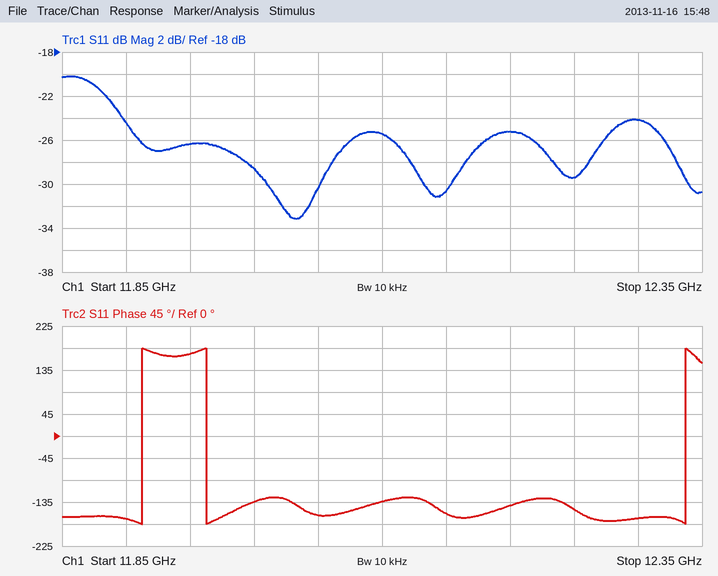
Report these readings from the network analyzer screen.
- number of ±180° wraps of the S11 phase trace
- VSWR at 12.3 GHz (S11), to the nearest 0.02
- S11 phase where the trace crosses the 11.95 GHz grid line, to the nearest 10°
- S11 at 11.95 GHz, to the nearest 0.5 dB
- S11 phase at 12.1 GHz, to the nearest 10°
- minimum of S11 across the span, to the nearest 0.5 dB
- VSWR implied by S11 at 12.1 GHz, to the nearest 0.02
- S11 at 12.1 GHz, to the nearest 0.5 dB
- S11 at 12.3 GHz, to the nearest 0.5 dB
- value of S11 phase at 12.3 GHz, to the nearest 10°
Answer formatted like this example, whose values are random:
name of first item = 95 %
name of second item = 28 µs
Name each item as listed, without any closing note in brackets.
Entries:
number of ±180° wraps of the S11 phase trace = 3
VSWR at 12.3 GHz (S11), to the nearest 0.02 = 1.14
S11 phase where the trace crosses the 11.95 GHz grid line, to the nearest 10° = 170°
S11 at 11.95 GHz, to the nearest 0.5 dB = -26.5 dB
S11 phase at 12.1 GHz, to the nearest 10° = -130°
minimum of S11 across the span, to the nearest 0.5 dB = -33.0 dB
VSWR implied by S11 at 12.1 GHz, to the nearest 0.02 = 1.12
S11 at 12.1 GHz, to the nearest 0.5 dB = -25.5 dB
S11 at 12.3 GHz, to the nearest 0.5 dB = -24.0 dB
value of S11 phase at 12.3 GHz, to the nearest 10° = -170°
